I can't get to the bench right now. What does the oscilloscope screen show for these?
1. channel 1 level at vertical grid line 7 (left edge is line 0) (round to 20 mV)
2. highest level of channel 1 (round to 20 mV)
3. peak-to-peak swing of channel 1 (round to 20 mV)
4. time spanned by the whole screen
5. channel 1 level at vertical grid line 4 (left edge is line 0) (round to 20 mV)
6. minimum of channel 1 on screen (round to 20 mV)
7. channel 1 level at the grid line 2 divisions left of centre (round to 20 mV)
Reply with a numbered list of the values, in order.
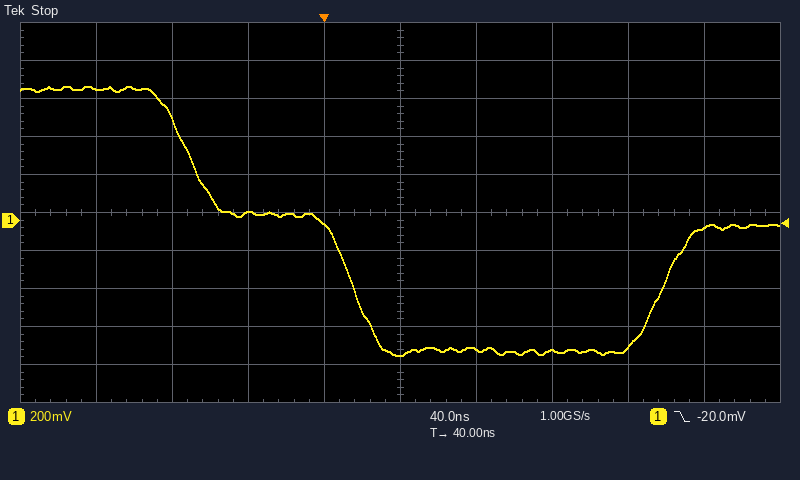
1. -680 mV
2. 700 mV
3. 1.42 V
4. 400 ns
5. -20 mV
6. -720 mV
7. 40 mV
